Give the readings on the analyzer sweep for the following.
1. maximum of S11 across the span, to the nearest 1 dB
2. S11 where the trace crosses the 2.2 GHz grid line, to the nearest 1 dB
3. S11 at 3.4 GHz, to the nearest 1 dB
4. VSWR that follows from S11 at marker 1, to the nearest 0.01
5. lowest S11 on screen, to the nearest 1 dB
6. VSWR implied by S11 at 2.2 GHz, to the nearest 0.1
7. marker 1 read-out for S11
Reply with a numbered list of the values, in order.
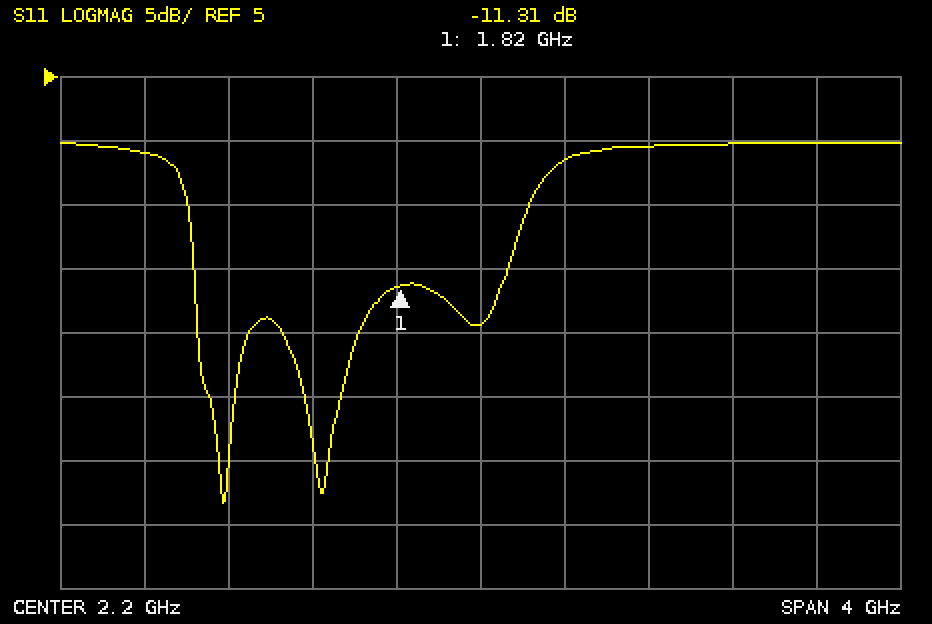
1. 0 dB
2. -14 dB
3. 0 dB
4. 1.75
5. -28 dB
6. 1.5
7. -11.31 dB
